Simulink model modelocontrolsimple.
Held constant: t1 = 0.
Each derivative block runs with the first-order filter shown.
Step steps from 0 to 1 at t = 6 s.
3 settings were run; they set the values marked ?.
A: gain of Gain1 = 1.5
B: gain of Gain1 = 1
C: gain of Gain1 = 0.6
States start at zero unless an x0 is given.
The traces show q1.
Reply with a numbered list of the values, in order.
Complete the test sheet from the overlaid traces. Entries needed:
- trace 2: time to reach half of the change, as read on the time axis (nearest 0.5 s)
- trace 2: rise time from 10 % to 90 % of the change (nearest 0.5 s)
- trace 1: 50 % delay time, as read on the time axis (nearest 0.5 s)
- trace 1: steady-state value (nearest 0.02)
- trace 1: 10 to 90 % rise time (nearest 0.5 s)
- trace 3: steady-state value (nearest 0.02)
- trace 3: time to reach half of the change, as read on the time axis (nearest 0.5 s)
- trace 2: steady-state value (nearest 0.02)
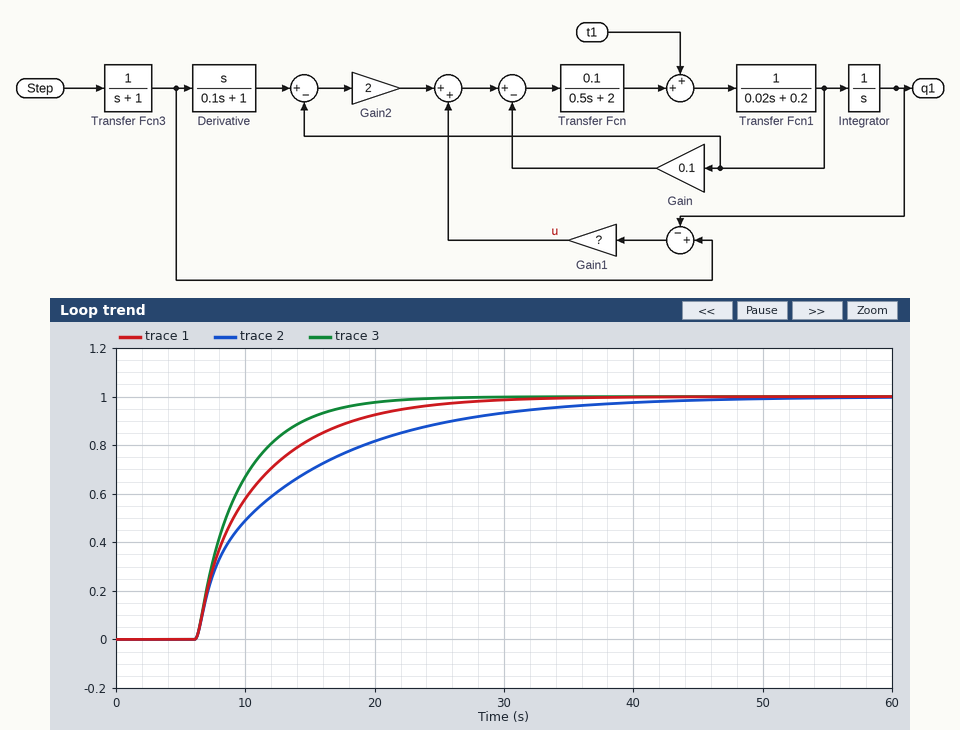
1. 10.0 s
2. 19.5 s
3. 9.0 s
4. 1.00
5. 11.5 s
6. 1.00
7. 8.5 s
8. 1.00
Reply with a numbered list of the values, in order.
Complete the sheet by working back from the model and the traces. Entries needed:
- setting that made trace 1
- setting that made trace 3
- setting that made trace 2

1. B
2. A
3. C
